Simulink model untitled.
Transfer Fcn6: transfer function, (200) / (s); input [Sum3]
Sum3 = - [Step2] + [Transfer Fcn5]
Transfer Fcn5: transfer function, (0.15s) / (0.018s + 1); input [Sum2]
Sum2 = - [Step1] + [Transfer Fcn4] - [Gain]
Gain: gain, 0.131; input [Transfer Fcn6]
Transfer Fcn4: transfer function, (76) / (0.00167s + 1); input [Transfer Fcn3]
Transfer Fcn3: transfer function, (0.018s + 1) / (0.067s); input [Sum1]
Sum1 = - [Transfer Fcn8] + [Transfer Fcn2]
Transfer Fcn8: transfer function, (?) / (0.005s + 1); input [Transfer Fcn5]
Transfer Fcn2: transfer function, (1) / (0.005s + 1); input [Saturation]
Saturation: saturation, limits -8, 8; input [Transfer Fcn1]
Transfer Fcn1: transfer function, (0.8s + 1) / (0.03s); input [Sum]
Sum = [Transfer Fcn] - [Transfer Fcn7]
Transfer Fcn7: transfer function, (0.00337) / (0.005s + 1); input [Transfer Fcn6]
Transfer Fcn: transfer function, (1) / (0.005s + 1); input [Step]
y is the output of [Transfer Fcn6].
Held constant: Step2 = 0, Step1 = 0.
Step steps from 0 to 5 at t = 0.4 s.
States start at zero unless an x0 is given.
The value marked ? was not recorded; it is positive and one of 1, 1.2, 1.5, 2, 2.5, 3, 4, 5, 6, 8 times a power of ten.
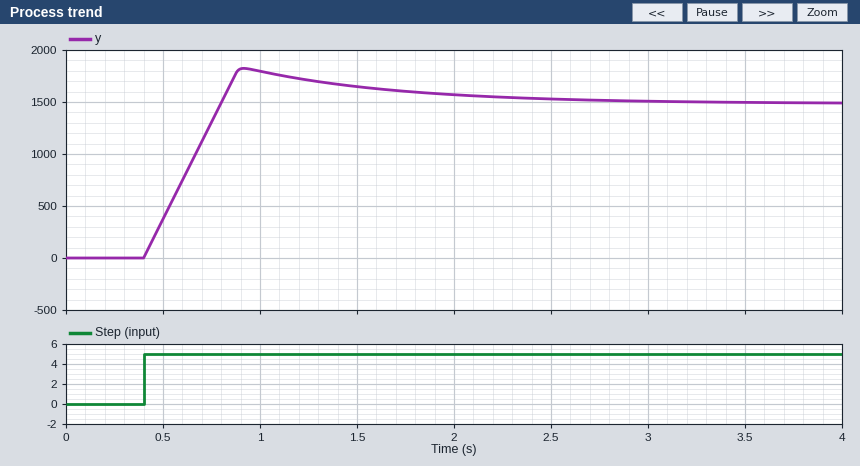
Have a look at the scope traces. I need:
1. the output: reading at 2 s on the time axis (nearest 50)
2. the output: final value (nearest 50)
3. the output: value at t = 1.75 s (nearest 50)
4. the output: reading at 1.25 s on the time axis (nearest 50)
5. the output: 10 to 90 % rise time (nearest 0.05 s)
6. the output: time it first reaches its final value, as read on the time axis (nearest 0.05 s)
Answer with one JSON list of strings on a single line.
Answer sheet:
["1550", "1500", "1600", "1700", "0.30 s", "0.80 s"]
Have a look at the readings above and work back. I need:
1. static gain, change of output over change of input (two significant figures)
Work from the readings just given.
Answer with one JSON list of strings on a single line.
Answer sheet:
["300"]
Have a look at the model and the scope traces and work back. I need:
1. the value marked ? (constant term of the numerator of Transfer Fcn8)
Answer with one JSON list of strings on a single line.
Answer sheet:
["0.4"]
